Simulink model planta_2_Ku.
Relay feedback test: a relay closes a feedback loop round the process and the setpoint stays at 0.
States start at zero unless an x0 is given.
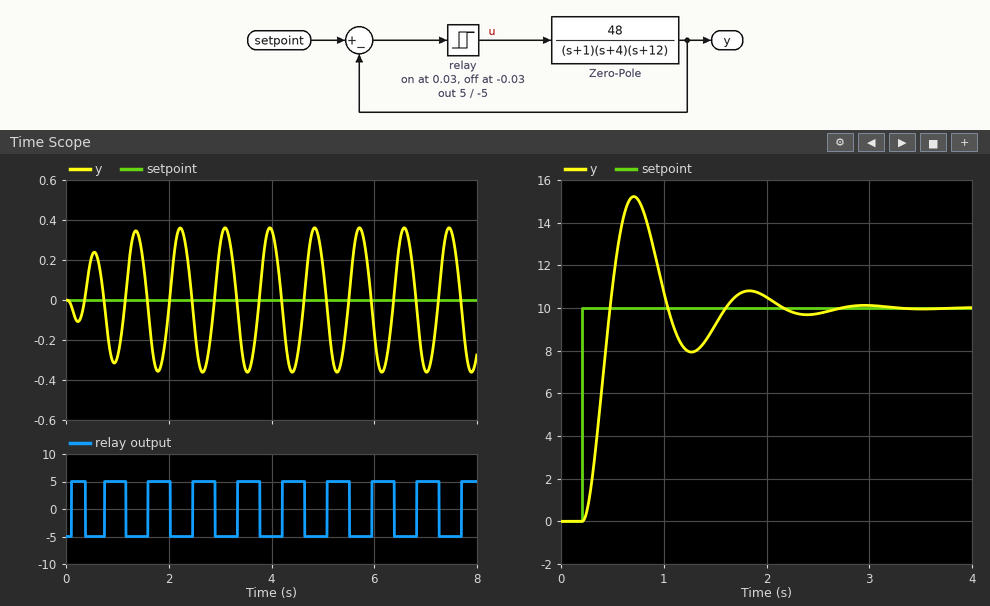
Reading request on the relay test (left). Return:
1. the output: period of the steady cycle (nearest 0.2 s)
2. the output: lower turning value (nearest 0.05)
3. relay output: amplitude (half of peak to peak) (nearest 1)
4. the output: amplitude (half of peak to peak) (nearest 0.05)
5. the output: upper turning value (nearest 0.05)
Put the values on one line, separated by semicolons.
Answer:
0.8 s; -0.35; 5; 0.35; 0.35
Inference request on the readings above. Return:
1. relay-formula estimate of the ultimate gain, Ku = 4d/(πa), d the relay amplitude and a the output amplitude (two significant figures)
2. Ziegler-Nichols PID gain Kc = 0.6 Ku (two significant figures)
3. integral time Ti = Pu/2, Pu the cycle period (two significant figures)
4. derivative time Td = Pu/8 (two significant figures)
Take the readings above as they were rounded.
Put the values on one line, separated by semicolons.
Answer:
18; 11; 0.40 s; 0.10 s
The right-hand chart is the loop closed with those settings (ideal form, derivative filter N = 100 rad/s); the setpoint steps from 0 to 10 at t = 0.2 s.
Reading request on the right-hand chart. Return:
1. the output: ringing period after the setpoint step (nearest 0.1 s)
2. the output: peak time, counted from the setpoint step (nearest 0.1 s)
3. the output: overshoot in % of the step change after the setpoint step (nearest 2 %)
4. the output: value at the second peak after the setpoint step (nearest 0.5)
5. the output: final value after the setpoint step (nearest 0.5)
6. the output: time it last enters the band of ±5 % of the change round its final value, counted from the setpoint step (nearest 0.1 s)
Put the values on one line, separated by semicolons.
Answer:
1.1 s; 0.5 s; 52 %; 11.0; 10.0; 1.8 s
